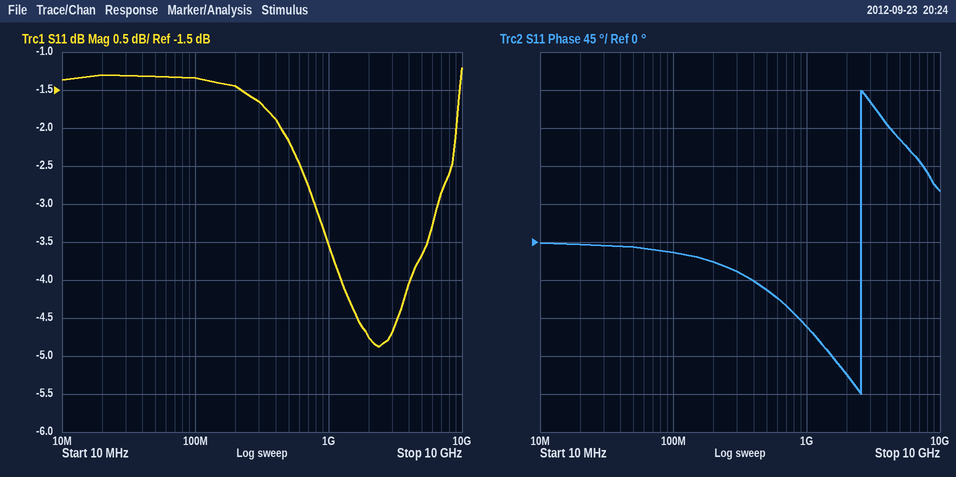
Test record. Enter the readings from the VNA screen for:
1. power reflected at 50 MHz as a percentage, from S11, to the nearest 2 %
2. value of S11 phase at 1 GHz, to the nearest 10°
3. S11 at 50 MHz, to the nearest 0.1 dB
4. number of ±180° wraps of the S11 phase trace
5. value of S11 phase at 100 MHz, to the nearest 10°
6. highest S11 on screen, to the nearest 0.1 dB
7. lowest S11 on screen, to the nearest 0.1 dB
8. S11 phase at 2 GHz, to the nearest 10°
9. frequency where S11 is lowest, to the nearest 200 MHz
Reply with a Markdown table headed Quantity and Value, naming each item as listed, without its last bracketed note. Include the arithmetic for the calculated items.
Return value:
| Quantity | Value |
|---|---|
| power reflected at 50 MHz as a percentage, from S11, to the nearest 2 % | 10^(-1.3/10) ≈ 74 % |
| value of S11 phase at 1 GHz, to the nearest 10° | -100° |
| S11 at 50 MHz, to the nearest 0.1 dB | -1.3 dB |
| number of ±180° wraps of the S11 phase trace | 1 |
| value of S11 phase at 100 MHz, to the nearest 10° | -10° |
| highest S11 on screen, to the nearest 0.1 dB | -1.2 dB |
| lowest S11 on screen, to the nearest 0.1 dB | -4.9 dB |
| S11 phase at 2 GHz, to the nearest 10° | -160° |
| frequency where S11 is lowest, to the nearest 200 MHz | 2.4 GHz |
